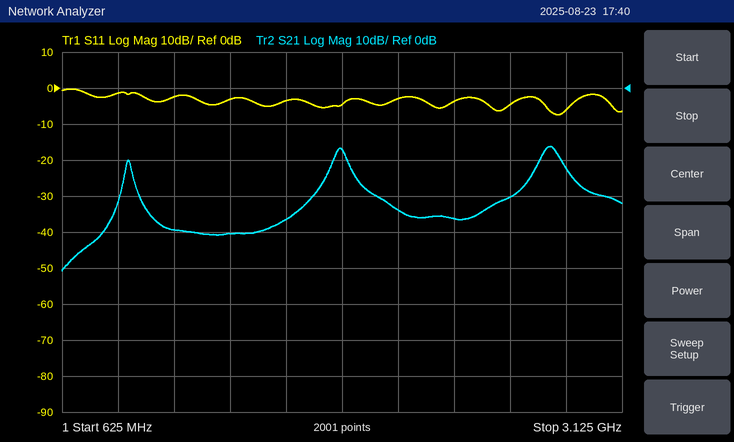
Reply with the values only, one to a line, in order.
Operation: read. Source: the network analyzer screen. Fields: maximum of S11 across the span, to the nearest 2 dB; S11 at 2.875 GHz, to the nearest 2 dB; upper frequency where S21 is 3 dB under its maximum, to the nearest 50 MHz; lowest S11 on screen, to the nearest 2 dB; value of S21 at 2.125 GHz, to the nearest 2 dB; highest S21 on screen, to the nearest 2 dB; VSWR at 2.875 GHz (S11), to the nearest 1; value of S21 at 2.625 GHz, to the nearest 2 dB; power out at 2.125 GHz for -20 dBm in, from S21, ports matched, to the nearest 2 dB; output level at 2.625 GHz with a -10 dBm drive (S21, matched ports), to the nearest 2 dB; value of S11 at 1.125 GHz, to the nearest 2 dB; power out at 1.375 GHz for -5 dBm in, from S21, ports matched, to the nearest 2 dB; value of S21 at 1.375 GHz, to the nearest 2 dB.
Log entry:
0 dB
-6 dB
2.85 GHz
-8 dB
-34 dB
-16 dB
3
-30 dB
-54 dBm
-40 dBm
-2 dB
-46 dBm
-40 dB
